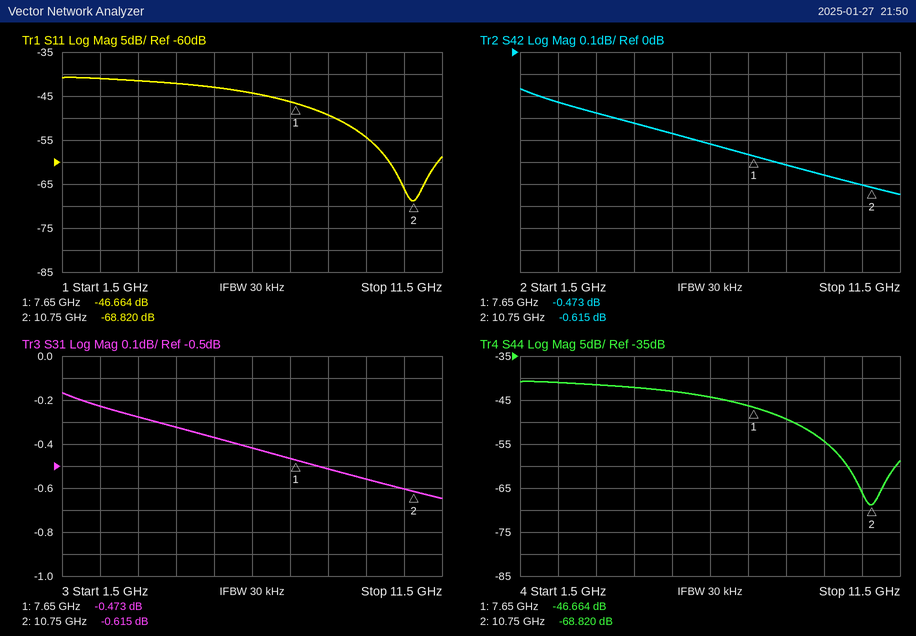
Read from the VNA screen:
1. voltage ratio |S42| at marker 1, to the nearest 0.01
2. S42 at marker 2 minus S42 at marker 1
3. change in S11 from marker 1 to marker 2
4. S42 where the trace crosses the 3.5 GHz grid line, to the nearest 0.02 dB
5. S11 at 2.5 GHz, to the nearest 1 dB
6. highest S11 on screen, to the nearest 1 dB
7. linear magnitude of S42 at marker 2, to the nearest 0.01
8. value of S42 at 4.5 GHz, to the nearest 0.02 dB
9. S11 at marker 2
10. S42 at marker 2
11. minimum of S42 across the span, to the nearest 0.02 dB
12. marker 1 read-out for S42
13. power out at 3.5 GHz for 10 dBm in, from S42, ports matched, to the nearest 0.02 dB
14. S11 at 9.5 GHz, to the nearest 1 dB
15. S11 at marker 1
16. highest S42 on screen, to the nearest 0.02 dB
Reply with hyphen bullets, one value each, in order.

- 0.95
- -0.142 dB
- -22.156 dB
- -0.28 dB
- -41 dB
- -41 dB
- 0.93
- -0.32 dB
- -68.820 dB
- -0.615 dB
- -0.64 dB
- -0.473 dB
- 9.72 dBm
- -54 dB
- -46.664 dB
- -0.16 dB
